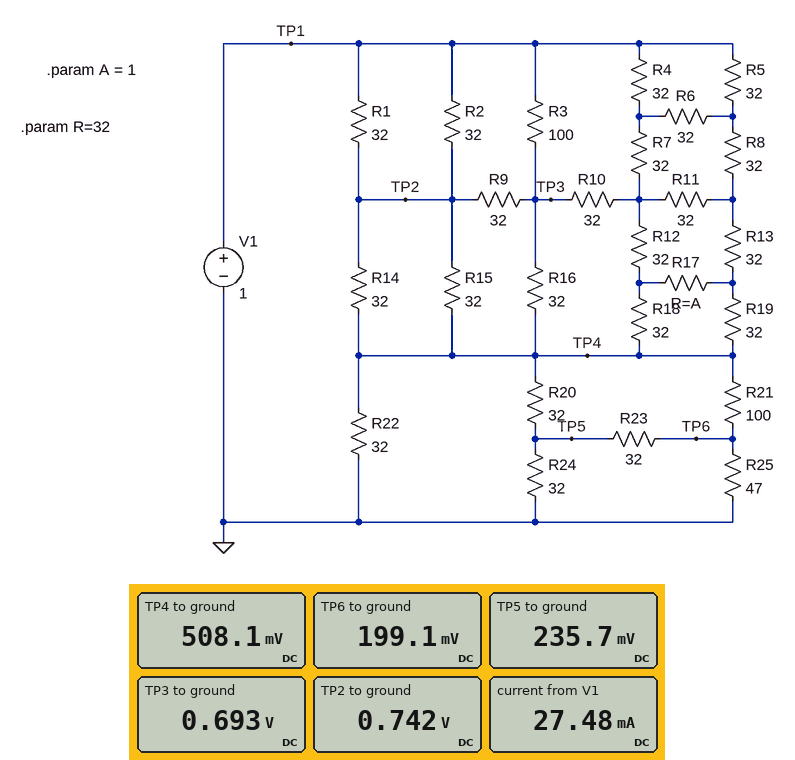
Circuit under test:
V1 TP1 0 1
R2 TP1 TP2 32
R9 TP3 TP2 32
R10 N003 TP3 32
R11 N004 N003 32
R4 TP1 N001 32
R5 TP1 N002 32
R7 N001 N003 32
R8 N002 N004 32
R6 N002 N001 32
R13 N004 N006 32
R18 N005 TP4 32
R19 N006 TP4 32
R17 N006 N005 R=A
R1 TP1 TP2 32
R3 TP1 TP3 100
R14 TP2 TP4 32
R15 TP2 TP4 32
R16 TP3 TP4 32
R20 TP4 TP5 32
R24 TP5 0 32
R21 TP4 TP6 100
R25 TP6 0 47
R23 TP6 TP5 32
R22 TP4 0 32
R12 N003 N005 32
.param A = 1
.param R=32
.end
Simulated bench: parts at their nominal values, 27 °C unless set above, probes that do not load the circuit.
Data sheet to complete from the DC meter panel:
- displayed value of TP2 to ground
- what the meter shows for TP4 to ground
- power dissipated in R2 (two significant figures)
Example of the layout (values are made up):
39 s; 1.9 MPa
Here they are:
0.742 V; 508.1 mV; 2.1 mW
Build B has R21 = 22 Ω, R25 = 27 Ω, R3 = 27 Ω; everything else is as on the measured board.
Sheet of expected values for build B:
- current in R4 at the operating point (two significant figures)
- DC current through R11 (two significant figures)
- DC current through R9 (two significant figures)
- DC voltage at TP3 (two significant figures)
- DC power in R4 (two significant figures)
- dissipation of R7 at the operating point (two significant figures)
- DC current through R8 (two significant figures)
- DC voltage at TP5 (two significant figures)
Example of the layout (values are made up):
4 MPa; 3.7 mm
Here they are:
3.9 mA; 68 µA; 330 µA; 760 mV; 500 µW; 490 µW; 4.0 mA; 250 mV
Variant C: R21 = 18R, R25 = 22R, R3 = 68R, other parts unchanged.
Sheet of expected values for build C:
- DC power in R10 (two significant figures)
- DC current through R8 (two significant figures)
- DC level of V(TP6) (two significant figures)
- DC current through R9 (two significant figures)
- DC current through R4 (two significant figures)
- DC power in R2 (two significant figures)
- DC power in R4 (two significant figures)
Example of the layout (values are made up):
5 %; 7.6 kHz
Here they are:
30 µW; 4.5 mA; 240 mV; 1.3 mA; 4.6 mA; 2.6 mW; 680 µW
